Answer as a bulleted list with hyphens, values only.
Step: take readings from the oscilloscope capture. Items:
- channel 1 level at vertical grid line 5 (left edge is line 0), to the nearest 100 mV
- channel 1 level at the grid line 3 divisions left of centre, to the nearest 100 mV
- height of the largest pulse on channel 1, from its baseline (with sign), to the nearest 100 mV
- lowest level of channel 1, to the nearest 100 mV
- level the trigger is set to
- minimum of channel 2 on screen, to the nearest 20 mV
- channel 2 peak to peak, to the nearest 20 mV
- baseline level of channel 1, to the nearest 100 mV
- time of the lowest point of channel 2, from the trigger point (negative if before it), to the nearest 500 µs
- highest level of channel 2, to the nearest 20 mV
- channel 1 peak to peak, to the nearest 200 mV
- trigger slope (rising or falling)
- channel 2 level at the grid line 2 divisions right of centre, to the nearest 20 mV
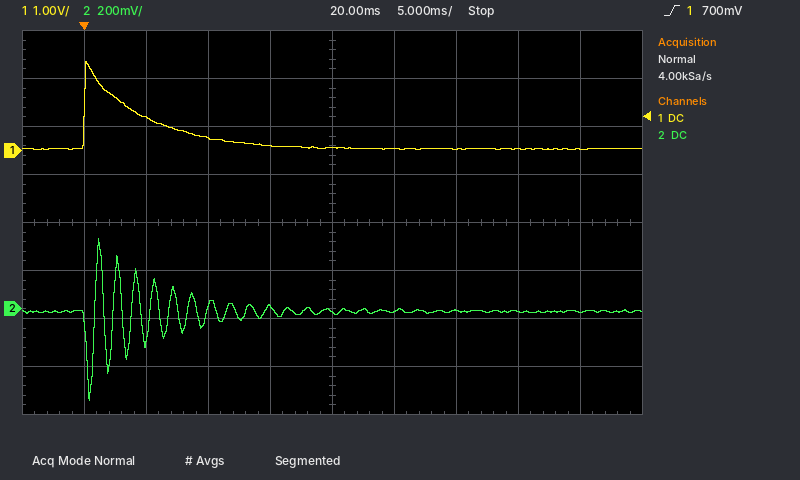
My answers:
- 100 mV
- 700 mV
- +1.8 V
- 0.0 V
- 700 mV
- -380 mV
- 680 mV
- 0.0 V
- +500 µs
- 300 mV
- 1.8 V
- rising
- 0 mV
